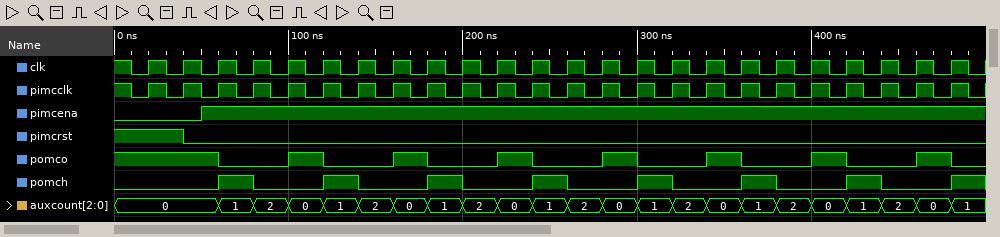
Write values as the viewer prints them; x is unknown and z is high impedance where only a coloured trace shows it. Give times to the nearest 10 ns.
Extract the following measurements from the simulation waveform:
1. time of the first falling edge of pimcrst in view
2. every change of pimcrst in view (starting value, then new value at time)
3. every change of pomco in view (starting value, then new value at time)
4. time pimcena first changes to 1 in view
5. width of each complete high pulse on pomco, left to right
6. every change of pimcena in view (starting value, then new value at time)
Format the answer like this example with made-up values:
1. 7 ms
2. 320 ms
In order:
1. 40 ns
2. 1, 0 at 40 ns
3. 1, 0 at 60 ns, 1 at 100 ns, 0 at 120 ns, 1 at 160 ns, 0 at 180 ns, 1 at 220 ns, 0 at 240 ns, 1 at 280 ns, 0 at 300 ns, 1 at 340 ns, 0 at 360 ns, 1 at 400 ns, 0 at 420 ns, 1 at 460 ns, 0 at 480 ns
4. 50 ns
5. 20 ns, 20 ns, 20 ns, 20 ns, 20 ns, 20 ns, 20 ns
6. 0, 1 at 50 ns
